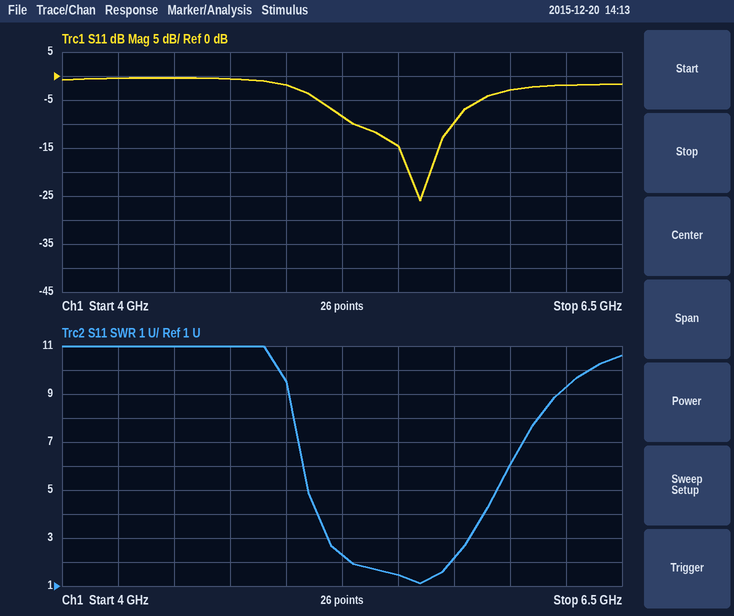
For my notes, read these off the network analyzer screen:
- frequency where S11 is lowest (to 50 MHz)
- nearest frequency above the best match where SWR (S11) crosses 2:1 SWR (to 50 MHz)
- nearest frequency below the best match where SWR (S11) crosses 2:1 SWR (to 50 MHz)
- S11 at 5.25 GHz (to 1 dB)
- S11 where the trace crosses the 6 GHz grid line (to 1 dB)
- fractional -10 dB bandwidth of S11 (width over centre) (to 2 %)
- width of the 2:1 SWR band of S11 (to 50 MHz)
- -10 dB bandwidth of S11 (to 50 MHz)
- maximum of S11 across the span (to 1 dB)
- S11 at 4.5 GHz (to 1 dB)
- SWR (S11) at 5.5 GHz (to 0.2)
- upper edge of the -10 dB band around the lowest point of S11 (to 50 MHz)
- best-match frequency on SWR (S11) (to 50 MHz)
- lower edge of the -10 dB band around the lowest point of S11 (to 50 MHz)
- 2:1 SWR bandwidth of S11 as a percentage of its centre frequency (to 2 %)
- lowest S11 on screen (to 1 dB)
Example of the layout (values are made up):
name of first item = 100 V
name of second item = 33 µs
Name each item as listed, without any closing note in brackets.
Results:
frequency where S11 is lowest = 5.60 GHz
nearest frequency above the best match where SWR (S11) crosses 2:1 SWR = 5.75 GHz
nearest frequency below the best match where SWR (S11) crosses 2:1 SWR = 5.30 GHz
S11 at 5.25 GHz = -8 dB
S11 where the trace crosses the 6 GHz grid line = -3 dB
fractional -10 dB bandwidth of S11 (width over centre) = 8 %
width of the 2:1 SWR band of S11 = 450 MHz
-10 dB bandwidth of S11 = 450 MHz
maximum of S11 across the span = 0 dB
S11 at 4.5 GHz = 0 dB
SWR (S11) at 5.5 GHz = 1.4
upper edge of the -10 dB band around the lowest point of S11 = 5.75 GHz
best-match frequency on SWR (S11) = 5.60 GHz
lower edge of the -10 dB band around the lowest point of S11 = 5.30 GHz
2:1 SWR bandwidth of S11 as a percentage of its centre frequency = 8 %
lowest S11 on screen = -26 dB
